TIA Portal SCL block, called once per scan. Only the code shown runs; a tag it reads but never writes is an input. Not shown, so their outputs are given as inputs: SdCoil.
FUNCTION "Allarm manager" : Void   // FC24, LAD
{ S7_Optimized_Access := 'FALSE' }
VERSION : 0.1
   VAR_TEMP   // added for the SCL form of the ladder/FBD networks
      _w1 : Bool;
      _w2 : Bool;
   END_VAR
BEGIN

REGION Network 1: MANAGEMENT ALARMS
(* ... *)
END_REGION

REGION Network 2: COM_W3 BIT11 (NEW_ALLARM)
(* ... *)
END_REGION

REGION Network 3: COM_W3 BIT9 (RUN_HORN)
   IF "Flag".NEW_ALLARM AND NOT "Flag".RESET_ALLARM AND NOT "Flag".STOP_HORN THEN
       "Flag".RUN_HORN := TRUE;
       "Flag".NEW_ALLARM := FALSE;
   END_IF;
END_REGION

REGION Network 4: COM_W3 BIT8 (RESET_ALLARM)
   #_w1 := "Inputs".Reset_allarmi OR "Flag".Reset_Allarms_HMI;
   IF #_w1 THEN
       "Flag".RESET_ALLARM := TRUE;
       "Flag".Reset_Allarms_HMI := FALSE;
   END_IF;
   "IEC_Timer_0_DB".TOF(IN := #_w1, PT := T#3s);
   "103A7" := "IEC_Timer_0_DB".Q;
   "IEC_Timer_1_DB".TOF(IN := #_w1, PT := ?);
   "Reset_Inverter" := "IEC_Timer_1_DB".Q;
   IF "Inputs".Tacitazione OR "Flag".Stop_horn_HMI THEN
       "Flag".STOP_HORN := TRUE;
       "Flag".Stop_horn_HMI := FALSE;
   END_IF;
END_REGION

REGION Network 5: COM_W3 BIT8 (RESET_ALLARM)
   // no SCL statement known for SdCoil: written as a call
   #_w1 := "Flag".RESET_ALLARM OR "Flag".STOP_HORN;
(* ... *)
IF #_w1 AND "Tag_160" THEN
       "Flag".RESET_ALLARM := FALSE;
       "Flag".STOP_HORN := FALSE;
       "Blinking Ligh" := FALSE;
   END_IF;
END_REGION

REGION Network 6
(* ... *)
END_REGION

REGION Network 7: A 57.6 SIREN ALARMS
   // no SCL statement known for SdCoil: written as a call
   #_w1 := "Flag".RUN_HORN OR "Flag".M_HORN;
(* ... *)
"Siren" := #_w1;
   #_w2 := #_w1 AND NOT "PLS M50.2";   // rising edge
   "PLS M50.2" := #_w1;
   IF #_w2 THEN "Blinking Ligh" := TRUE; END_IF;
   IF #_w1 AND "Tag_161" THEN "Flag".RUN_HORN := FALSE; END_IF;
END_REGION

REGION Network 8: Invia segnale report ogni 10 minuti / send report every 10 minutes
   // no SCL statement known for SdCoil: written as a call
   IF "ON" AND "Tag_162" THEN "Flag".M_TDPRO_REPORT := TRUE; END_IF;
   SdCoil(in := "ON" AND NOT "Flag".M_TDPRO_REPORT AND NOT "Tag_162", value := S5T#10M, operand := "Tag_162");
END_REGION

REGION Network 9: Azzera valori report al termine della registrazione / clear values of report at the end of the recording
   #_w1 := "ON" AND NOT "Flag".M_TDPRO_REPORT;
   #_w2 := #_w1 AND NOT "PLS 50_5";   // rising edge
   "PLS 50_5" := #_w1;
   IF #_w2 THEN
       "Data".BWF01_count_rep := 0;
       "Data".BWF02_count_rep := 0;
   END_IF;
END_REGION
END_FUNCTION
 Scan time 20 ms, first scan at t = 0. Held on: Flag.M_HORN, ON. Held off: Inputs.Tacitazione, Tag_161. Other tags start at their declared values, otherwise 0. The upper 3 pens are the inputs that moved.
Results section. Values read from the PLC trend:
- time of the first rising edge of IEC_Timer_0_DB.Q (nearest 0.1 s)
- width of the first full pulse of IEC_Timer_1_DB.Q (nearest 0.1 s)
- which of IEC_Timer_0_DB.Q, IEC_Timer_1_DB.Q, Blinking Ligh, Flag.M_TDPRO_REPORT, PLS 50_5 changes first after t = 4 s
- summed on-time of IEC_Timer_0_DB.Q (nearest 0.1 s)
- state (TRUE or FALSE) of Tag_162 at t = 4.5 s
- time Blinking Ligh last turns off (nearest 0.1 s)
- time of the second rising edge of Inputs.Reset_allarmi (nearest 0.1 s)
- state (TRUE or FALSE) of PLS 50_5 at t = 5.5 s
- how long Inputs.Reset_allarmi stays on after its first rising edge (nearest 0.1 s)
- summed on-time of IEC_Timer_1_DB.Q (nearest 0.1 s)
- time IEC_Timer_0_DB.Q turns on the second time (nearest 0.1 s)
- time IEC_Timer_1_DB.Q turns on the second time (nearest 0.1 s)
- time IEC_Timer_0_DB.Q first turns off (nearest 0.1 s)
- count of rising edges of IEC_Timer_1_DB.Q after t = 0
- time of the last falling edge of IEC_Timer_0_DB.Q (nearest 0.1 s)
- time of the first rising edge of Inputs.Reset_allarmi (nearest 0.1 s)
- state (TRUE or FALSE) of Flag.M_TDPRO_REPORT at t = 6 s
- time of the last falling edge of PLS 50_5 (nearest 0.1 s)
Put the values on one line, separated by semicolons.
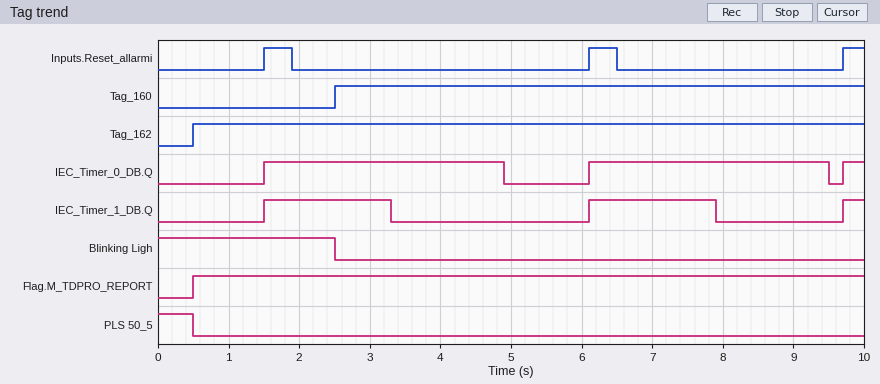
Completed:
1.5 s; 1.8 s; IEC_Timer_0_DB.Q; 7.1 s; TRUE; 2.5 s; 6.1 s; FALSE; 0.4 s; 3.9 s; 6.1 s; 6.1 s; 4.9 s; 3; 9.5 s; 1.5 s; TRUE; 0.5 s
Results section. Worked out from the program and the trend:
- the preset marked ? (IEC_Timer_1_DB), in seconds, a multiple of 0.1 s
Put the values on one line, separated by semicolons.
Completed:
1.4 s
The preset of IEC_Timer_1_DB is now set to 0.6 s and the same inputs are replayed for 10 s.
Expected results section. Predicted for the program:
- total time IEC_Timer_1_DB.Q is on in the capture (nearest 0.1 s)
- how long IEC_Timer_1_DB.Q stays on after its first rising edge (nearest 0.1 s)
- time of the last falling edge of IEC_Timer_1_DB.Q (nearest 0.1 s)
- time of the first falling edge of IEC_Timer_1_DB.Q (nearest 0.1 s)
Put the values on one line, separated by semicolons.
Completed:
2.3 s; 1.0 s; 7.1 s; 2.5 s
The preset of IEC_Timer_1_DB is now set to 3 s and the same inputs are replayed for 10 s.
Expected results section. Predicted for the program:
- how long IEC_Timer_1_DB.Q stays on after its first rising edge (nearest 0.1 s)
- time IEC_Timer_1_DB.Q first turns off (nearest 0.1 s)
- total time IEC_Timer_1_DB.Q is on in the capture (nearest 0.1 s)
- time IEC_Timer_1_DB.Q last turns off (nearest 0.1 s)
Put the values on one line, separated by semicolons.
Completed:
3.4 s; 4.9 s; 7.1 s; 9.5 s
